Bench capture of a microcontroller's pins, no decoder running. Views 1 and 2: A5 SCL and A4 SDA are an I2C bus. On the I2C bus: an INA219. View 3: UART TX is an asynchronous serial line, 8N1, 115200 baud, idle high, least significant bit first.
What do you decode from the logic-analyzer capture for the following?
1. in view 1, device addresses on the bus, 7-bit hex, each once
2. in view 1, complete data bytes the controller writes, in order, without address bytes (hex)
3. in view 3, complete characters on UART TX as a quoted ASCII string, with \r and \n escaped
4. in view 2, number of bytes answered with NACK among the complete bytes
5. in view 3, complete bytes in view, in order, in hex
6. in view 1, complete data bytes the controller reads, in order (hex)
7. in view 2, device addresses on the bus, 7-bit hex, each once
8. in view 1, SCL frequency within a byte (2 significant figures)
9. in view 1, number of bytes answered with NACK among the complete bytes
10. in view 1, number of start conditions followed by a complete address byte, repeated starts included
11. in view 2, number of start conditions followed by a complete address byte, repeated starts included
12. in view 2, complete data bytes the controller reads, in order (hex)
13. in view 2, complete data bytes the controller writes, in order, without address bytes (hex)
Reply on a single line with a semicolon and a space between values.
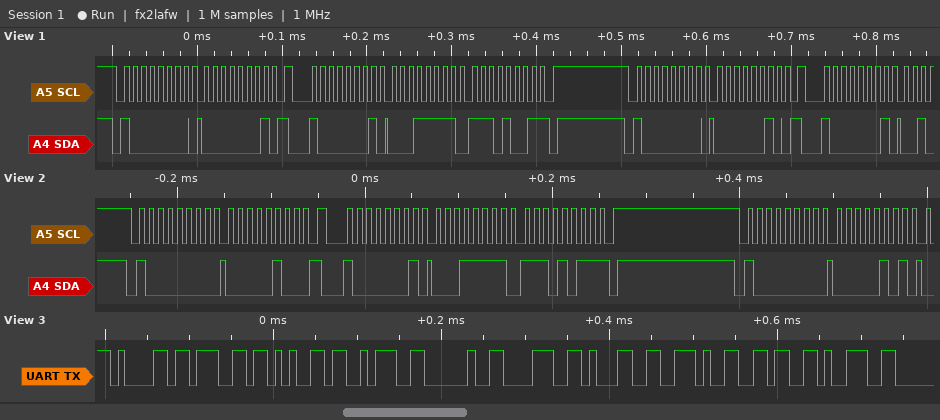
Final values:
0x40; 01 02; "age: 81.69"; 1; 0x61 0x67 0x65 0x3A 0x20 0x38 0x31 0x2E 0x36 0x39; 1F E9; 0x40; 100 kHz; 1; 4; 3; 1F EB; 04 05
